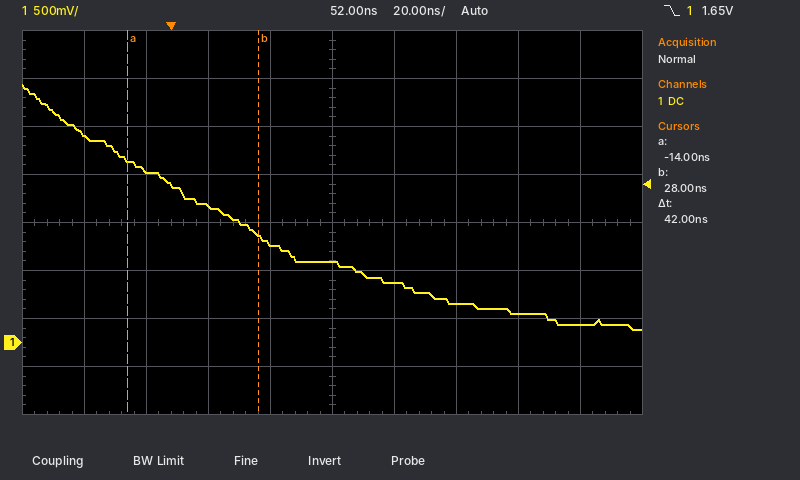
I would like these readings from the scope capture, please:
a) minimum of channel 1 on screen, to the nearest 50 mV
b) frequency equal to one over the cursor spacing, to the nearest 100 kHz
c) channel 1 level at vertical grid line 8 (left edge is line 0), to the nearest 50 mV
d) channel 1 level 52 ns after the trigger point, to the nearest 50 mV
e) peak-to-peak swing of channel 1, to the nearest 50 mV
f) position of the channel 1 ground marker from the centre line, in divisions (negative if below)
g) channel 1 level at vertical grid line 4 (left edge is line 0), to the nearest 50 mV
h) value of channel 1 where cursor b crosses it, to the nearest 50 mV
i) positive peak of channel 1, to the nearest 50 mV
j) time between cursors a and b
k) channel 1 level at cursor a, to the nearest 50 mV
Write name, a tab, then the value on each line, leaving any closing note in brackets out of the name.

minimum of channel 1 on screen, to the nearest 50 mV	150 mV
frequency equal to one over the cursor spacing, to the nearest 100 kHz	23.8 MHz
channel 1 level at vertical grid line 8 (left edge is line 0), to the nearest 50 mV	300 mV
channel 1 level 52 ns after the trigger point, to the nearest 50 mV	850 mV
peak-to-peak swing of channel 1, to the nearest 50 mV	2.55 V
position of the channel 1 ground marker from the centre line, in divisions	-2.5 div
channel 1 level at vertical grid line 4 (left edge is line 0), to the nearest 50 mV	1.05 V
value of channel 1 where cursor b crosses it, to the nearest 50 mV	1.10 V
positive peak of channel 1, to the nearest 50 mV	2.70 V
time between cursors a and b	42 ns
channel 1 level at cursor a, to the nearest 50 mV	1.90 V
